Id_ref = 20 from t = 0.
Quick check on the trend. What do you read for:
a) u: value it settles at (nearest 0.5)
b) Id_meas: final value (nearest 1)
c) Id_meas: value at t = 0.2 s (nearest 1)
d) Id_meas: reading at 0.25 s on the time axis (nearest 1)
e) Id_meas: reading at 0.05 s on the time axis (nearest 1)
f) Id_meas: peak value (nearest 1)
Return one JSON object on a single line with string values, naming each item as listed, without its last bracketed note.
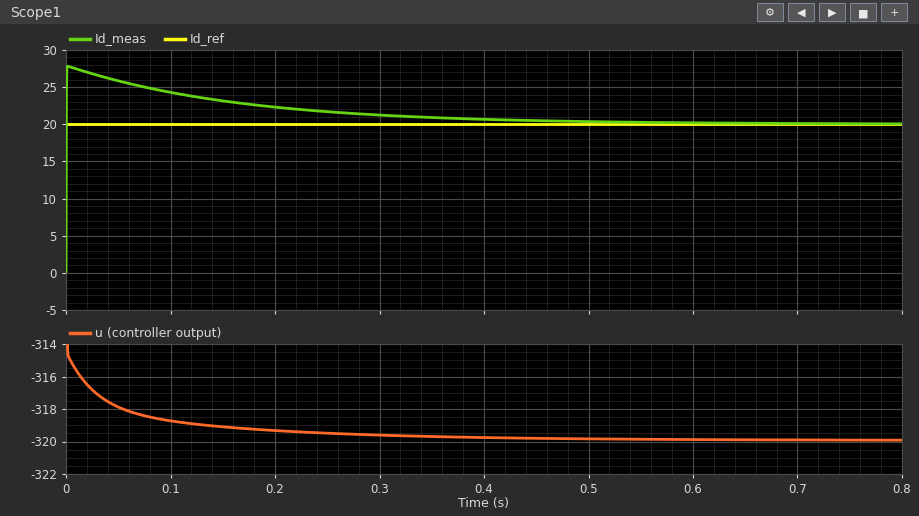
{"u: value it settles at": "-320.0", "Id_meas: final value": "20", "Id_meas: value at t = 0.2 s": "22", "Id_meas: reading at 0.25 s on the time axis": "22", "Id_meas: reading at 0.05 s on the time axis": "26", "Id_meas: peak value": "28"}
